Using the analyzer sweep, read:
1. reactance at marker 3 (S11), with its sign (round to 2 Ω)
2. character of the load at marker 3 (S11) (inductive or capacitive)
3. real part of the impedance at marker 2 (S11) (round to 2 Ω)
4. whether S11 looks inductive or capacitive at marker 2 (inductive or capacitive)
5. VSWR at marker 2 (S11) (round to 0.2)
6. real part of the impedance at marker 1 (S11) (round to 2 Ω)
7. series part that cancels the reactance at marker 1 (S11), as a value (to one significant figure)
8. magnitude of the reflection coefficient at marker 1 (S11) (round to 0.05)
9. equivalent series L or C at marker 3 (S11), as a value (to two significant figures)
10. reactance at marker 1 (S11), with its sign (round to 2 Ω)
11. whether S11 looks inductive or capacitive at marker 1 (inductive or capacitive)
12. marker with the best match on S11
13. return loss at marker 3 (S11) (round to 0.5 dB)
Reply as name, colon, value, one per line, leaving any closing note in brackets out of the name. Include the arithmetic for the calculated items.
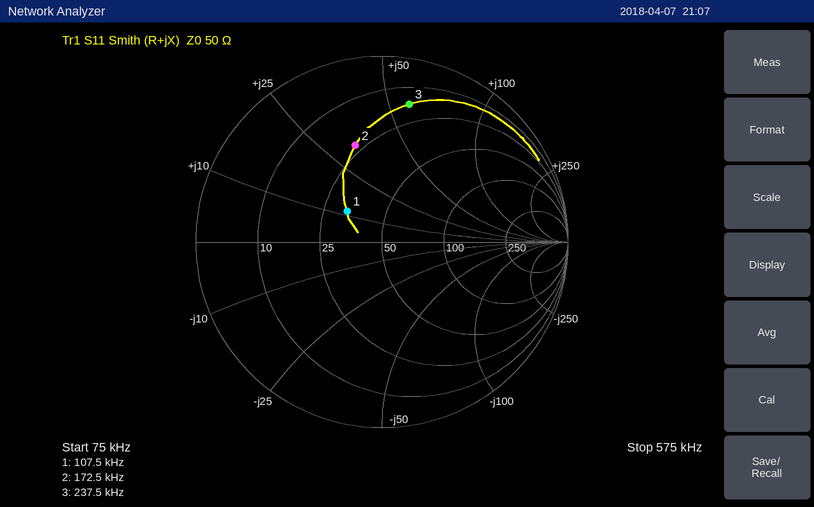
reactance at marker 3 (S11), with its sign: +58 Ω
character of the load at marker 3 (S11): inductive
real part of the impedance at marker 2 (S11): 22 Ω
whether S11 looks inductive or capacitive at marker 2: inductive
VSWR at marker 2 (S11): 3.4
real part of the impedance at marker 1 (S11): 32 Ω
series part that cancels the reactance at marker 1 (S11), as a value: C = 1/(2π × 107.5 kHz × 12 Ω) ≈ 123 nF, so 100 nF to one significant figure
magnitude of the reflection coefficient at marker 1 (S11): 0.25
equivalent series L or C at marker 3 (S11), as a value: L = 58 Ω/(2π × 237.5 kHz) ≈ 39 µH
reactance at marker 1 (S11), with its sign: +12 Ω
whether S11 looks inductive or capacitive at marker 1: inductive
marker with the best match on S11: marker 1
return loss at marker 3 (S11): 2.5 dB
